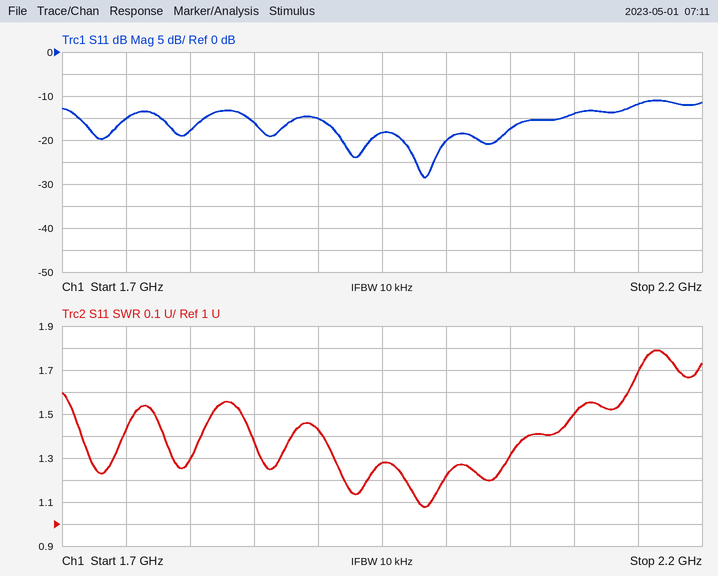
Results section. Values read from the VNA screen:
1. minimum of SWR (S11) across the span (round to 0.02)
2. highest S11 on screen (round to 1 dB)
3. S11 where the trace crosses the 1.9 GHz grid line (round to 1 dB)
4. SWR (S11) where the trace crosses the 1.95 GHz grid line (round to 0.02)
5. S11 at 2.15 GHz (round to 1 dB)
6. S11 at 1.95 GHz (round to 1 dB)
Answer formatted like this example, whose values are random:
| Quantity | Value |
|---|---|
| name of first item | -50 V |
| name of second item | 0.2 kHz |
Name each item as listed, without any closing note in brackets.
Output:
| Quantity | Value |
|---|---|
| minimum of SWR (S11) across the span | 1.08 |
| highest S11 on screen | -11 dB |
| S11 where the trace crosses the 1.9 GHz grid line | -15 dB |
| SWR (S11) where the trace crosses the 1.95 GHz grid line | 1.28 |
| S11 at 2.15 GHz | -12 dB |
| S11 at 1.95 GHz | -18 dB |
